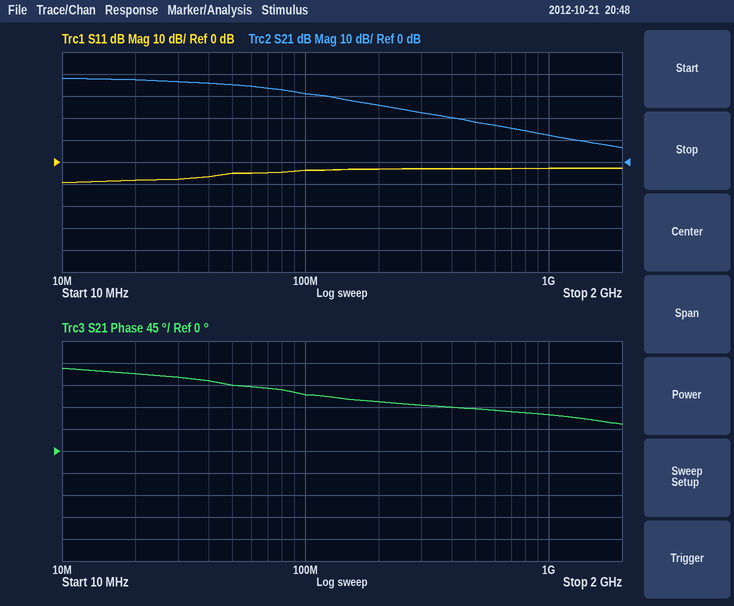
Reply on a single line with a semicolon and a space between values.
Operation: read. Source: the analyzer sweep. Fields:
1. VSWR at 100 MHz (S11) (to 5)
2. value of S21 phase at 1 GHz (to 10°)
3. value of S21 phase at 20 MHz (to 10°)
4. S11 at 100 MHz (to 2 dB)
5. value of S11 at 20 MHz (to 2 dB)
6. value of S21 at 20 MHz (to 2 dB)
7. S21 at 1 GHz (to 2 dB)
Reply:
5; 70°; 160°; -4 dB; -8 dB; 38 dB; 12 dB
